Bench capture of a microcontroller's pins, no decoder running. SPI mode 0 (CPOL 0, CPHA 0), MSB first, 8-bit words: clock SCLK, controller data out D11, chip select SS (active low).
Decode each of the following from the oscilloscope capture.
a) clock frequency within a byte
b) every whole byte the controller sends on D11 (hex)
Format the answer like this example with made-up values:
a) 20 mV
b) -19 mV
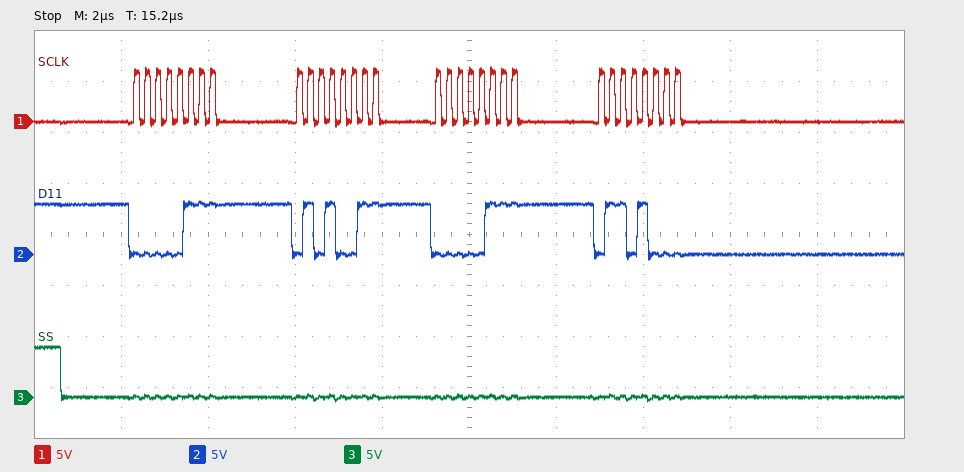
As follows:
a) 4 MHz
b) 07 53 07 68
